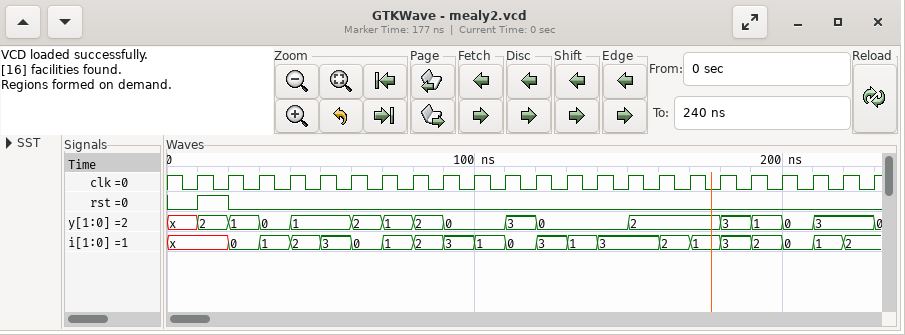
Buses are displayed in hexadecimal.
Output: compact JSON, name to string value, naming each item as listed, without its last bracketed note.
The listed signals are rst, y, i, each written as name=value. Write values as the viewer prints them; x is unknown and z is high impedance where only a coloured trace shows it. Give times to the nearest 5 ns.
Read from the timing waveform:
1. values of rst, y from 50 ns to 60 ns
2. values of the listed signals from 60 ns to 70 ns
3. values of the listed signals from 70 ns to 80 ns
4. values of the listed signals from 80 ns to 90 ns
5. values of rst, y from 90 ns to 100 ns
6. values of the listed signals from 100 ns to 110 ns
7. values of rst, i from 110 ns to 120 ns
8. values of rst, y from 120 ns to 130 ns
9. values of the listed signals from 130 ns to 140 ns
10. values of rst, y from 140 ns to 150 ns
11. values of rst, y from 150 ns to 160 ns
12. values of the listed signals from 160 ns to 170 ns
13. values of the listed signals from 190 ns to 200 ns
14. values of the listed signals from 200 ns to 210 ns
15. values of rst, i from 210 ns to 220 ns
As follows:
{"values of rst, y from 50 ns to 60 ns": "rst=0, y=1", "values of the listed signals from 60 ns to 70 ns": "rst=0, y=2, i=0", "values of the listed signals from 70 ns to 80 ns": "rst=0, y=1, i=1", "values of the listed signals from 80 ns to 90 ns": "rst=0, y=2, i=2", "values of rst, y from 90 ns to 100 ns": "rst=0, y=0", "values of the listed signals from 100 ns to 110 ns": "rst=0, y=0, i=1", "values of rst, i from 110 ns to 120 ns": "rst=0, i=0", "values of rst, y from 120 ns to 130 ns": "rst=0, y=0", "values of the listed signals from 130 ns to 140 ns": "rst=0, y=0, i=1", "values of rst, y from 140 ns to 150 ns": "rst=0, y=0", "values of rst, y from 150 ns to 160 ns": "rst=0, y=2", "values of the listed signals from 160 ns to 170 ns": "rst=0, y=2, i=2", "values of the listed signals from 190 ns to 200 ns": "rst=0, y=1, i=2", "values of the listed signals from 200 ns to 210 ns": "rst=0, y=0, i=0", "values of rst, i from 210 ns to 220 ns": "rst=0, i=1"}
